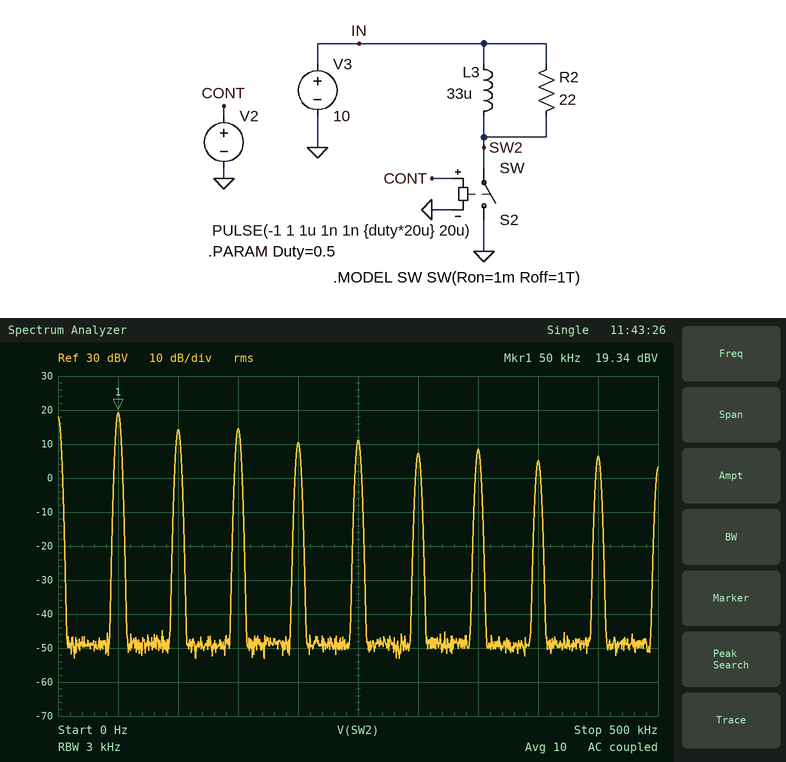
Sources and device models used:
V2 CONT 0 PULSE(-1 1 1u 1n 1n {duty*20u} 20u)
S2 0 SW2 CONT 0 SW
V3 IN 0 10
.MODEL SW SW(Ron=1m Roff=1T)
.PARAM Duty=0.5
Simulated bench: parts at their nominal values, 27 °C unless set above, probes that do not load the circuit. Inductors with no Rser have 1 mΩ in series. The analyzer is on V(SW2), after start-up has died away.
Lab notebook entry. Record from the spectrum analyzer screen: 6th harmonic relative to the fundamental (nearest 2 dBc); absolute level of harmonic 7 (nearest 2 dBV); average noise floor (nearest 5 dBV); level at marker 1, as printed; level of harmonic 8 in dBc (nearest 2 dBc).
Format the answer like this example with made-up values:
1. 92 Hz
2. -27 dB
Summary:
1. -12 dBc
2. 8 dBV
3. -50 dBV
4. 19.34 dBV
5. -14 dBc
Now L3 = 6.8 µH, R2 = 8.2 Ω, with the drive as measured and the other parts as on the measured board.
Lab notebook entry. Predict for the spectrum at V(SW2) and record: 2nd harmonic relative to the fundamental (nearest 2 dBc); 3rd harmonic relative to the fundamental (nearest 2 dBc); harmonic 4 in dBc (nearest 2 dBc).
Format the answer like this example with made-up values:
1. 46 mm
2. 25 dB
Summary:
1. -4 dBc
2. -2 dBc
3. -6 dBc
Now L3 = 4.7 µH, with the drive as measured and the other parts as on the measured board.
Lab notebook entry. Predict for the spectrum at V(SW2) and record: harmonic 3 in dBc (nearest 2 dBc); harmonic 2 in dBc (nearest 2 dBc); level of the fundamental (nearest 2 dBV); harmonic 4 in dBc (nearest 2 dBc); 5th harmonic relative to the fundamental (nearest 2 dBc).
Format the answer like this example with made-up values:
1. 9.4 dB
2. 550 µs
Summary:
1. -2 dBc
2. -2 dBc
3. 18 dBV
4. -2 dBc
5. -2 dBc
